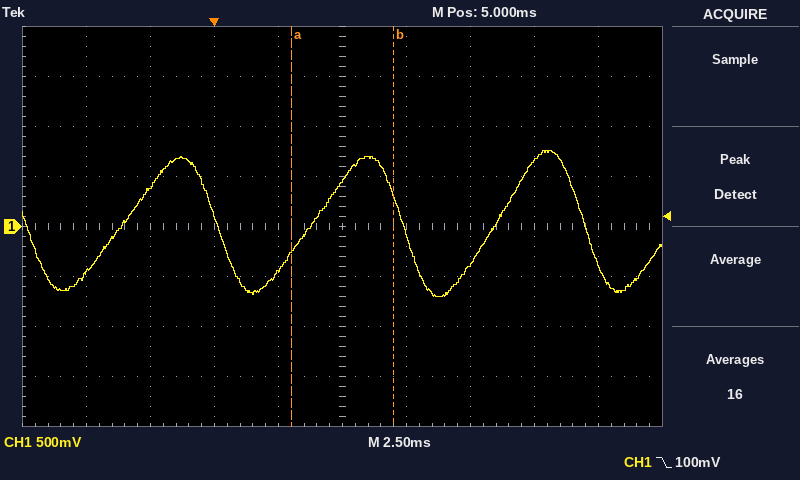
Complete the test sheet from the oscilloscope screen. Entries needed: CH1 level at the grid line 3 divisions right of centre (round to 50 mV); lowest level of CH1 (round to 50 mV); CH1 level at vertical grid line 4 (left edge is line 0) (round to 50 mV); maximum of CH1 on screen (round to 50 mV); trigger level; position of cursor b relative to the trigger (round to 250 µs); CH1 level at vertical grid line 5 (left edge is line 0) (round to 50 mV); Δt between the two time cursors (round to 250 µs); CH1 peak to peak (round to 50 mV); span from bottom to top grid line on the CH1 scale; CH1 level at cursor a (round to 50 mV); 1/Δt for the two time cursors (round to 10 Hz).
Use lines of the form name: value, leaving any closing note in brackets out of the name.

CH1 level at the grid line 3 divisions right of centre: 650 mV
lowest level of CH1: -700 mV
CH1 level at vertical grid line 4 (left edge is line 0): -450 mV
maximum of CH1 on screen: 750 mV
trigger level: 100 mV
position of cursor b relative to the trigger: +7.00 ms
CH1 level at vertical grid line 5 (left edge is line 0): 450 mV
Δt between the two time cursors: 4.00 ms
CH1 peak to peak: 1.45 V
span from bottom to top grid line on the CH1 scale: 4 V
CH1 level at cursor a: -250 mV
1/Δt for the two time cursors: 250 Hz
